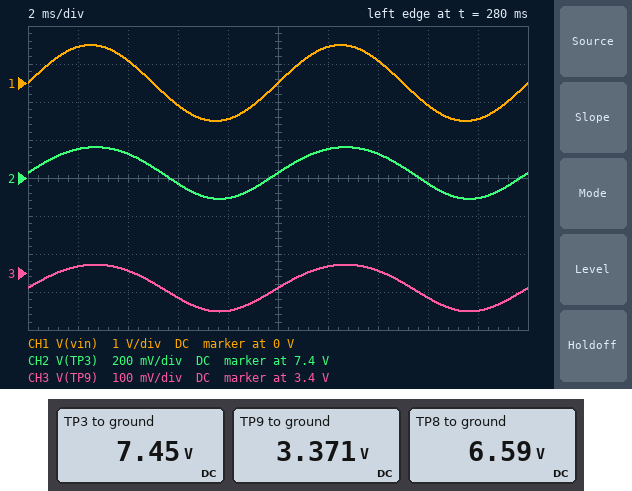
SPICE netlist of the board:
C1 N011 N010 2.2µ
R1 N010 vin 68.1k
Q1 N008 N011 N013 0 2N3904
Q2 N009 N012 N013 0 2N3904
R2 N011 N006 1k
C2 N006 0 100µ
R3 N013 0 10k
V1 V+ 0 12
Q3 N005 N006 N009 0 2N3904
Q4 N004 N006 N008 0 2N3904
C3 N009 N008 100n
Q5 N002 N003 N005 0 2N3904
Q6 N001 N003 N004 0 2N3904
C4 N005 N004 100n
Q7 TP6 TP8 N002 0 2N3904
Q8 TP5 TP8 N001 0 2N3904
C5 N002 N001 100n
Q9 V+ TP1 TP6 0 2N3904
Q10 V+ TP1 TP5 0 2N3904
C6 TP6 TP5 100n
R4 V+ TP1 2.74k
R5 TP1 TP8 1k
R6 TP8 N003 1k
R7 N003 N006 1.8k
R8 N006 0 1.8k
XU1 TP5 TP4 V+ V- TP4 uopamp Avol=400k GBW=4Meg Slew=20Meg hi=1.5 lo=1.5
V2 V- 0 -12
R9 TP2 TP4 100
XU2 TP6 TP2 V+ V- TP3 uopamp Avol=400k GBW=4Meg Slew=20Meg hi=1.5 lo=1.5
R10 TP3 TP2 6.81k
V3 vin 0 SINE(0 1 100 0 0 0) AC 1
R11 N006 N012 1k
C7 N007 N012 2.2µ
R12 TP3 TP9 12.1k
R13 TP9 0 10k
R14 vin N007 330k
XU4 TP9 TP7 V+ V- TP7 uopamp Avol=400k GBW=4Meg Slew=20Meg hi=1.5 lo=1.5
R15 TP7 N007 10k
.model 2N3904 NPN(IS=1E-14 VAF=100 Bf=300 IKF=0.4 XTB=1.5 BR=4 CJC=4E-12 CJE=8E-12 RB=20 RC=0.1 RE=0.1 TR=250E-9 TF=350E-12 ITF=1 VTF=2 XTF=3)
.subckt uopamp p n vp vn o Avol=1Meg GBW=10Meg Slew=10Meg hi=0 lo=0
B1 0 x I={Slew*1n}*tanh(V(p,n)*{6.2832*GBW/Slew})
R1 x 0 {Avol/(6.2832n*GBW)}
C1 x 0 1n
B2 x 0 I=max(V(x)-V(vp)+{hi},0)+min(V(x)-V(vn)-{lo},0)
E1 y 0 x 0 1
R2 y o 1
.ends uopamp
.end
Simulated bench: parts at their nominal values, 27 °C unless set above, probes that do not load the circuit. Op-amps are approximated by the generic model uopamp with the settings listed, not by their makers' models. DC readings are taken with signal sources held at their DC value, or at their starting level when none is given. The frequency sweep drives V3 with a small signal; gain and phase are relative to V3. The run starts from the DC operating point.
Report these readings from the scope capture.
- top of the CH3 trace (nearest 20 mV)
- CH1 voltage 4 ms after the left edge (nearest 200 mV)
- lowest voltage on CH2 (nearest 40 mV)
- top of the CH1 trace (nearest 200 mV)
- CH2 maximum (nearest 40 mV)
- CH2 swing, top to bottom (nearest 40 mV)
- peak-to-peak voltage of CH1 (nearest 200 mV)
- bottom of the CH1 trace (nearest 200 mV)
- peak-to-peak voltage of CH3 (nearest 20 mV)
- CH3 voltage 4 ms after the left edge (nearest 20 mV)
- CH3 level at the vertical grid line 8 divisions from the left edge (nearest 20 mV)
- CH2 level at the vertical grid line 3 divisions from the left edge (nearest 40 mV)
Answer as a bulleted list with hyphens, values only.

- 3.42 V
- 600 mV
- 7.28 V
- 1.0 V
- 7.56 V
- 280 mV
- 2.0 V
- -1.0 V
- 120 mV
- 3.40 V
- 3.34 V
- 7.36 V
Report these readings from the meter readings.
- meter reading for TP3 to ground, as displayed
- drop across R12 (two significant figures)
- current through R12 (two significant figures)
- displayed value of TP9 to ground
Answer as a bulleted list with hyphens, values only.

- 7.45 V
- 4.1 V
- 340 µA
- 3.371 V
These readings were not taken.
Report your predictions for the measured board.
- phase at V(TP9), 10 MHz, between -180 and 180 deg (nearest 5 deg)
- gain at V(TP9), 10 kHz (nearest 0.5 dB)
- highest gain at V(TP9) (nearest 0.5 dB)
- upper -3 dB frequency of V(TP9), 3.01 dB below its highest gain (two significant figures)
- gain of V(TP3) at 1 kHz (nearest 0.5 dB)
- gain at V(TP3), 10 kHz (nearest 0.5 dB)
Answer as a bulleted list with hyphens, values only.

- -85 deg
- -59.5 dB
- -19.0 dB
- 8.0 Hz
- -16.5 dB
- -52.5 dB
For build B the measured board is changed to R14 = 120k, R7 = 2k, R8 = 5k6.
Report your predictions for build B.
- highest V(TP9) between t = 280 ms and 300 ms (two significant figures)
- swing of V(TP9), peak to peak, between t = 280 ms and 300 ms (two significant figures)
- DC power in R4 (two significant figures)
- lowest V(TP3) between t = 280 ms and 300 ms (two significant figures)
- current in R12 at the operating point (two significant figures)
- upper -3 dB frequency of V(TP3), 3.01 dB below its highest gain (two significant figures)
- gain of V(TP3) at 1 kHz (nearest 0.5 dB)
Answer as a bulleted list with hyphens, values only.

- 3.9 V
- 65 mV
- 2.7 mW
- 8.6 V
- 390 µA
- 6.8 Hz
- -23.0 dB
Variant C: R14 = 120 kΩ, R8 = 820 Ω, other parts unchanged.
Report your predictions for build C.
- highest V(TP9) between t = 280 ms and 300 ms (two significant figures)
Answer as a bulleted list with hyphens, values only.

- 3.2 V
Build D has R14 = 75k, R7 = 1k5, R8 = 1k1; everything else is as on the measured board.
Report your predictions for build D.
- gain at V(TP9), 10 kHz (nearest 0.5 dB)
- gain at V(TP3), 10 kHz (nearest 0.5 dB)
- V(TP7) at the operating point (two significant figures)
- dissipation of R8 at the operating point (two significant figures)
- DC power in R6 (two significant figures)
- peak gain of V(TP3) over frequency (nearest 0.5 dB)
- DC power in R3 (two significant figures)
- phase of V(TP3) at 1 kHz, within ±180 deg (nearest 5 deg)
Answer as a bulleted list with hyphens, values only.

- -63.5 dB
- -56.5 dB
- 3.1 V
- 2.9 mW
- 2.7 mW
- -12.0 dB
- 140 µW
- -85 deg
